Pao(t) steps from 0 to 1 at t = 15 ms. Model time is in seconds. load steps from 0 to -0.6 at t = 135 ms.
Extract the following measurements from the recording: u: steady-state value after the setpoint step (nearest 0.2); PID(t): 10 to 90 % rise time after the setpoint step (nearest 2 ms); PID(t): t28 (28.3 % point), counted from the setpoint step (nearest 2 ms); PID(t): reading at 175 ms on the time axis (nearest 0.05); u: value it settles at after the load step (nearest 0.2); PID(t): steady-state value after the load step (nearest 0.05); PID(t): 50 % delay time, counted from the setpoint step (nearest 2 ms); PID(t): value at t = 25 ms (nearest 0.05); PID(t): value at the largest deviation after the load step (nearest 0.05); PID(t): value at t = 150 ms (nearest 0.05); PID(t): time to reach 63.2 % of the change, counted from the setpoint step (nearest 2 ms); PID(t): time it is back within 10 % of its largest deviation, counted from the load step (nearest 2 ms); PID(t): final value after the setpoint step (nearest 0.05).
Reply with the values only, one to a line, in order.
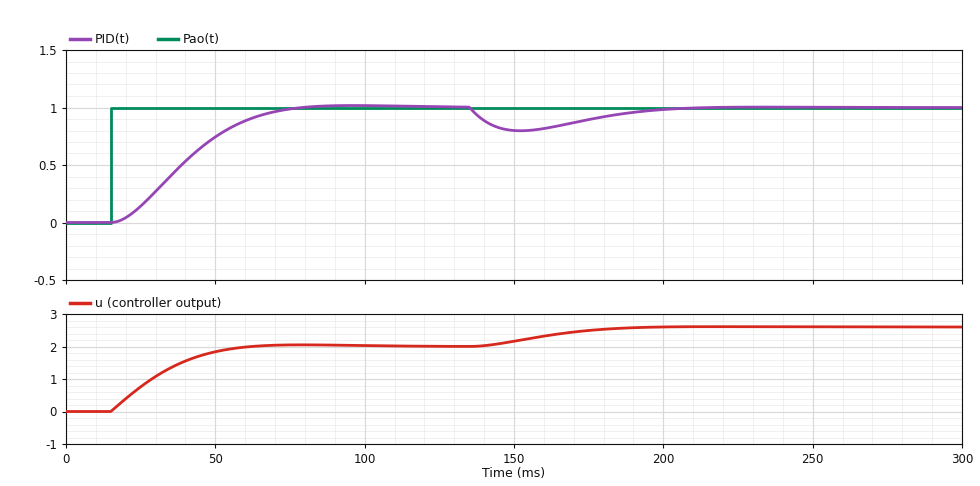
2.0
38 ms
16 ms
0.90
2.6
1.00
24 ms
0.15
0.80
0.80
30 ms
64 ms
1.00
